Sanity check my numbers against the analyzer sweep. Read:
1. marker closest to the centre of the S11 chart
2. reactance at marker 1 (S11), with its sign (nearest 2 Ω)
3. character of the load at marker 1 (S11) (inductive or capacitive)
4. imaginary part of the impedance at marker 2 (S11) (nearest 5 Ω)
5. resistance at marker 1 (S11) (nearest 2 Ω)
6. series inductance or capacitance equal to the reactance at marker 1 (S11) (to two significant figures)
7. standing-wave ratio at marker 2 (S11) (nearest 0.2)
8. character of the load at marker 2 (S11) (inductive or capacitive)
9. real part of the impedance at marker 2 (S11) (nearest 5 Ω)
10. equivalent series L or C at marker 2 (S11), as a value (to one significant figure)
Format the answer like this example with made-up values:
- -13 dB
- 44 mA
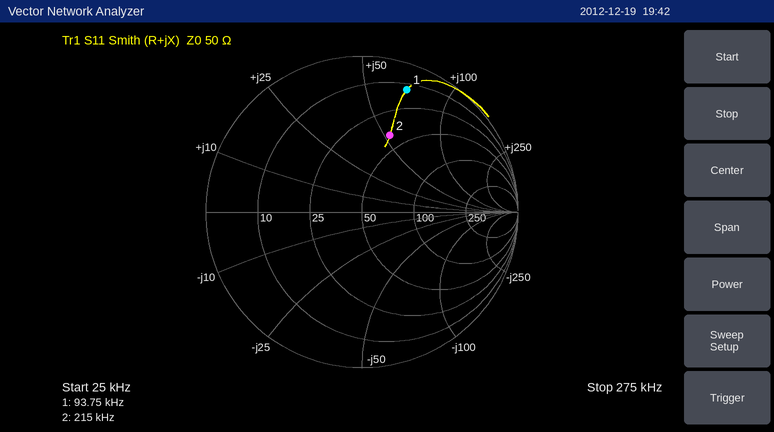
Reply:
- marker 2
- +70 Ω
- inductive
- +55 Ω
- 14 Ω
- 120 µH
- 3.2
- inductive
- 40 Ω
- 40 µH
